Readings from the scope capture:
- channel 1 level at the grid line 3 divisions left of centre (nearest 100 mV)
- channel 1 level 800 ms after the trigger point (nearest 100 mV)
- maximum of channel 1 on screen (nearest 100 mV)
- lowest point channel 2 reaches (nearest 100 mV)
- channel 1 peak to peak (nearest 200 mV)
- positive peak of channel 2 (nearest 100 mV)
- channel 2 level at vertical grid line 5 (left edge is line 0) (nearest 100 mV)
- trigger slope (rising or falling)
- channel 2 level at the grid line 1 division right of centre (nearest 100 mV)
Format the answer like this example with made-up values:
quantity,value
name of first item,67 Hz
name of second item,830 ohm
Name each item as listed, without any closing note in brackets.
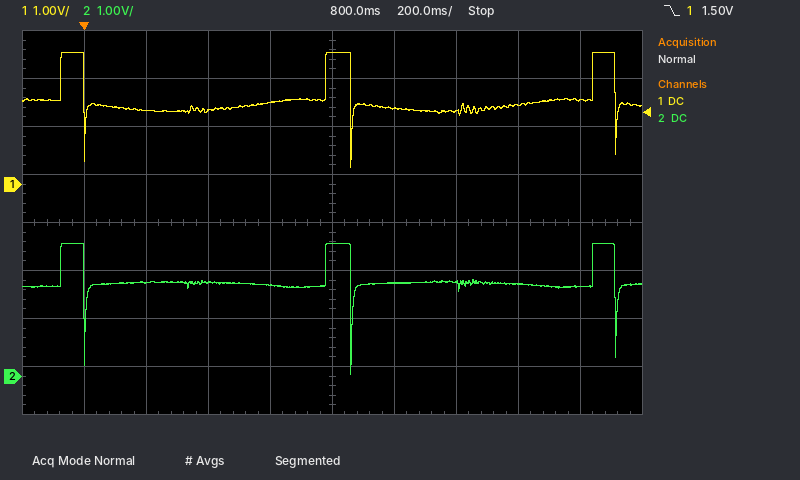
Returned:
quantity,value
channel 1 level at the grid line 3 divisions left of centre,1.5 V
channel 1 level 800 ms after the trigger point,2.7 V
maximum of channel 1 on screen,2.7 V
lowest point channel 2 reaches,0.0 V
channel 1 peak to peak,2.4 V
positive peak of channel 2,2.8 V
channel 2 level at vertical grid line 5 (left edge is line 0),2.8 V
trigger slope,falling
channel 2 level at the grid line 1 division right of centre,1.9 V
